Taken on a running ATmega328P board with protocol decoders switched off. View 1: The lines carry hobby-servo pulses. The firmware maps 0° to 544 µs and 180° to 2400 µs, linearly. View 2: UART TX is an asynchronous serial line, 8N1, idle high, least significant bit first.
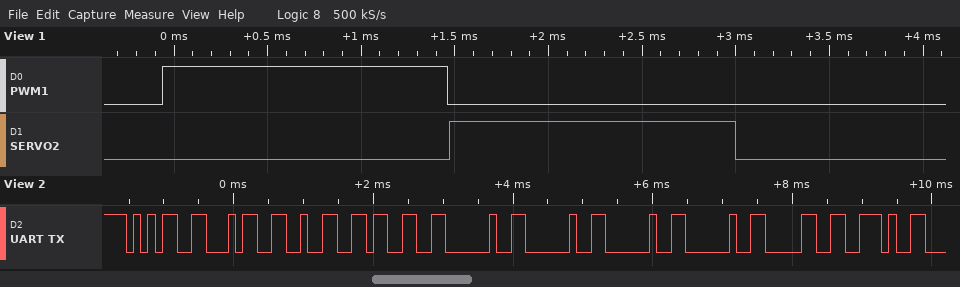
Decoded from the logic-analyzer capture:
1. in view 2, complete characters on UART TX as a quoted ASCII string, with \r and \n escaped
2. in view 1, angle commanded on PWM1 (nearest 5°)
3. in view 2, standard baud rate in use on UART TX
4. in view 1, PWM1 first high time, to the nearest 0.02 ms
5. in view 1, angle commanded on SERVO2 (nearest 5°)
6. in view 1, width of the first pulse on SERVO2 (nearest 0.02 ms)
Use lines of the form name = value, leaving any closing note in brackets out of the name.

in view 2, complete characters on UART TX as a quoted ASCII string, with \r and \n escaped = "5423    0."
in view 1, angle commanded on PWM1 = 95°
in view 2, standard baud rate in use on UART TX = 9600 baud
in view 1, PWM1 first high time, to the nearest 0.02 ms = 1.52 ms
in view 1, angle commanded on SERVO2 = 95°
in view 1, width of the first pulse on SERVO2 = 1.52 ms
